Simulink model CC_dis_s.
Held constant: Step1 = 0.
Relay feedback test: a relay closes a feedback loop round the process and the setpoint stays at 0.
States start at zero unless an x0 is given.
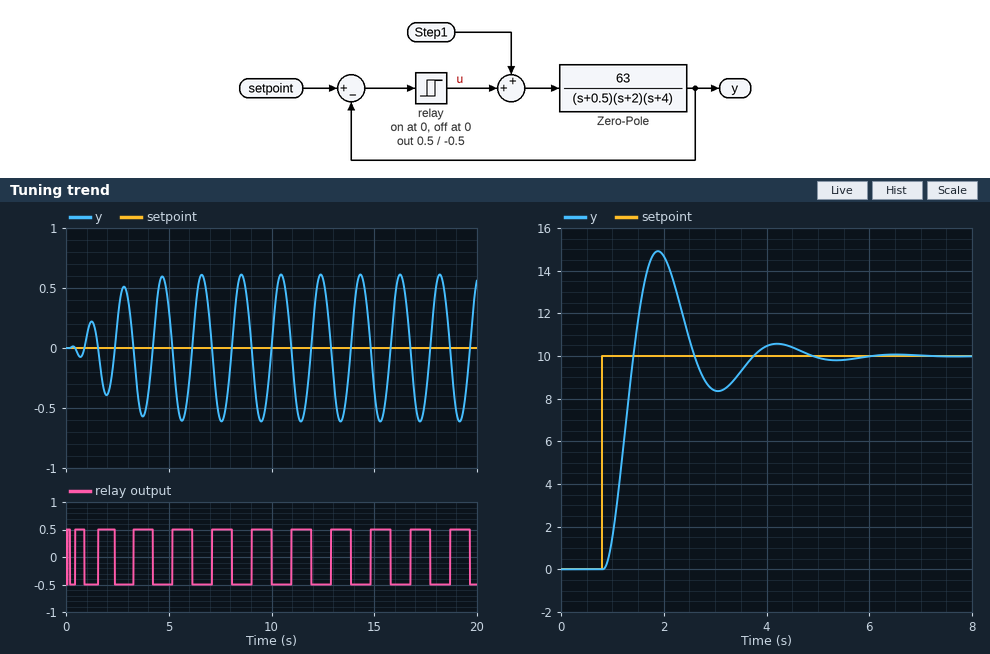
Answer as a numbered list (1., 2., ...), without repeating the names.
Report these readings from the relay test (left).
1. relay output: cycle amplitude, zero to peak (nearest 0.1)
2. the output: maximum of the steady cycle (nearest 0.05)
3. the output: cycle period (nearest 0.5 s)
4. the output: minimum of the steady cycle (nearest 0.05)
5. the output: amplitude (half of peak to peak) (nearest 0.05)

1. 0.5
2. 0.60
3. 2.0 s
4. -0.60
5. 0.60
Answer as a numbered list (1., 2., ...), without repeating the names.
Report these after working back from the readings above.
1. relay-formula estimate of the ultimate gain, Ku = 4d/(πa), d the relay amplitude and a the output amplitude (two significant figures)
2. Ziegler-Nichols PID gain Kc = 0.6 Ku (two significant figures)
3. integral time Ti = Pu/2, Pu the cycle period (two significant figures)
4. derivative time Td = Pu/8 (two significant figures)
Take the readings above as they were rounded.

1. 1.1
2. 0.66
3. 1.0 s
4. 0.25 s
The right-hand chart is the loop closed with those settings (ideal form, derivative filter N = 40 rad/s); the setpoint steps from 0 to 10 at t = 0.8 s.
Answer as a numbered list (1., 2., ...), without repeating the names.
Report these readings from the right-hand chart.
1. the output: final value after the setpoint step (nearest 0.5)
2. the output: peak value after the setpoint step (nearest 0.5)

1. 10.0
2. 15.0
